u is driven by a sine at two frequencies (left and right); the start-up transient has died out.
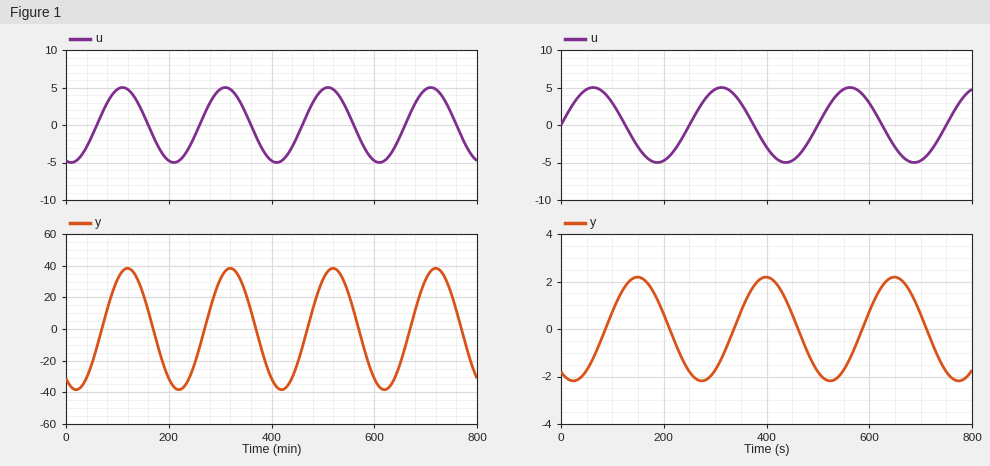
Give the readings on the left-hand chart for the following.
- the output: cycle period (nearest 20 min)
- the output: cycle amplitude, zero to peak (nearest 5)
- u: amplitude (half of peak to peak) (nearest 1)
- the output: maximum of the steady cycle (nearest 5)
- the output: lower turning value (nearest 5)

200 min
40
5
40
-40
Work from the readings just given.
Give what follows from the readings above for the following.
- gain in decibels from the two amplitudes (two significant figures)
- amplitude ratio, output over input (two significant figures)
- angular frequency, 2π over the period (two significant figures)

18 dB
8.0
0.031 rad/min
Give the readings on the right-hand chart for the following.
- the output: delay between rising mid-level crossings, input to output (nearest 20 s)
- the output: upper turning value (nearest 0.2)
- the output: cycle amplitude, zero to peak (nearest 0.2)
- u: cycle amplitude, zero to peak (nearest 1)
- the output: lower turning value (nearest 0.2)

80 s
2.2
2.2
5
-2.2
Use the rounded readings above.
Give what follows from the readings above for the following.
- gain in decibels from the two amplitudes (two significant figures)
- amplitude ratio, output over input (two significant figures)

-7.1 dB
0.44
